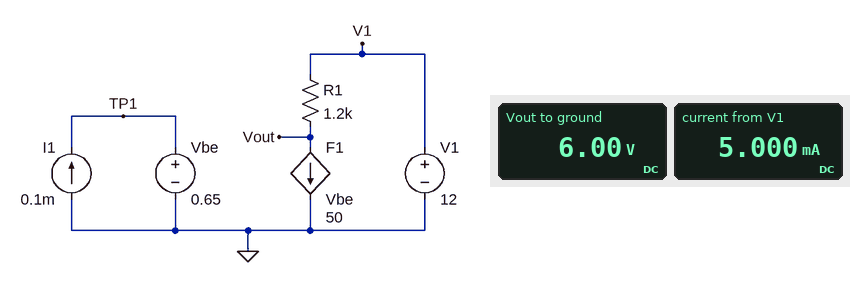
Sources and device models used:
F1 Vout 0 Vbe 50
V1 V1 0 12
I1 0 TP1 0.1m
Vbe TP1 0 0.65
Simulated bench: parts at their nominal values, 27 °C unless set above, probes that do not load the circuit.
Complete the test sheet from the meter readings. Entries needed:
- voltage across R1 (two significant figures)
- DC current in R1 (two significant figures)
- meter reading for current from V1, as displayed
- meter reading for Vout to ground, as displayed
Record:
6.0 V
5.0 mA
5.000 mA
6.00 V
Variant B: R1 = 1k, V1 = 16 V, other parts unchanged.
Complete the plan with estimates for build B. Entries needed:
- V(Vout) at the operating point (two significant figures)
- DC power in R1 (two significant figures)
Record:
11 V
25 mW
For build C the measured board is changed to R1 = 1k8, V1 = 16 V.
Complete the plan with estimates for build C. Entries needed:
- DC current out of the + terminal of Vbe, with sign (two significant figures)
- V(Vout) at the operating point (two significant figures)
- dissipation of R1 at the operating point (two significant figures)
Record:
-100 µA
7.0 V
45 mW
